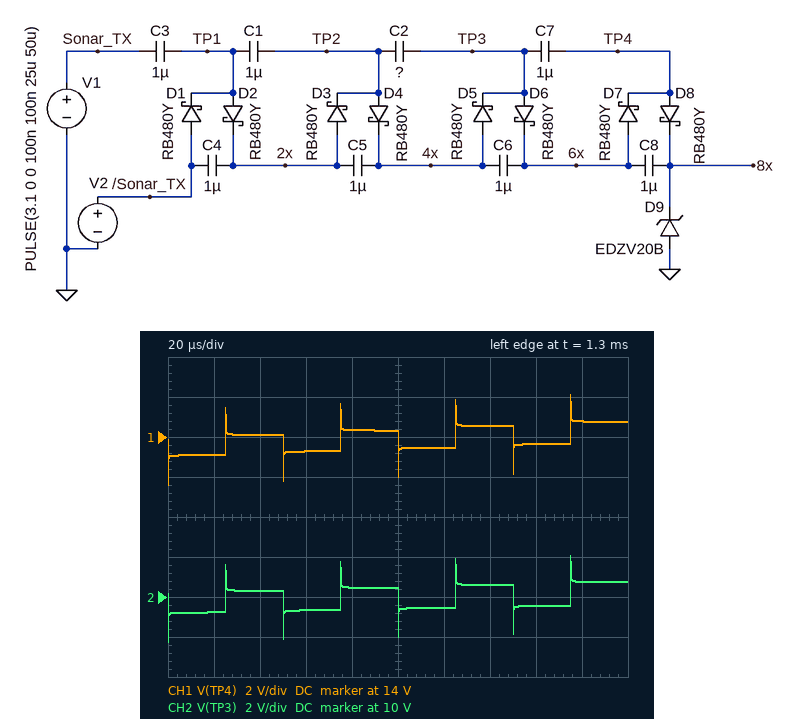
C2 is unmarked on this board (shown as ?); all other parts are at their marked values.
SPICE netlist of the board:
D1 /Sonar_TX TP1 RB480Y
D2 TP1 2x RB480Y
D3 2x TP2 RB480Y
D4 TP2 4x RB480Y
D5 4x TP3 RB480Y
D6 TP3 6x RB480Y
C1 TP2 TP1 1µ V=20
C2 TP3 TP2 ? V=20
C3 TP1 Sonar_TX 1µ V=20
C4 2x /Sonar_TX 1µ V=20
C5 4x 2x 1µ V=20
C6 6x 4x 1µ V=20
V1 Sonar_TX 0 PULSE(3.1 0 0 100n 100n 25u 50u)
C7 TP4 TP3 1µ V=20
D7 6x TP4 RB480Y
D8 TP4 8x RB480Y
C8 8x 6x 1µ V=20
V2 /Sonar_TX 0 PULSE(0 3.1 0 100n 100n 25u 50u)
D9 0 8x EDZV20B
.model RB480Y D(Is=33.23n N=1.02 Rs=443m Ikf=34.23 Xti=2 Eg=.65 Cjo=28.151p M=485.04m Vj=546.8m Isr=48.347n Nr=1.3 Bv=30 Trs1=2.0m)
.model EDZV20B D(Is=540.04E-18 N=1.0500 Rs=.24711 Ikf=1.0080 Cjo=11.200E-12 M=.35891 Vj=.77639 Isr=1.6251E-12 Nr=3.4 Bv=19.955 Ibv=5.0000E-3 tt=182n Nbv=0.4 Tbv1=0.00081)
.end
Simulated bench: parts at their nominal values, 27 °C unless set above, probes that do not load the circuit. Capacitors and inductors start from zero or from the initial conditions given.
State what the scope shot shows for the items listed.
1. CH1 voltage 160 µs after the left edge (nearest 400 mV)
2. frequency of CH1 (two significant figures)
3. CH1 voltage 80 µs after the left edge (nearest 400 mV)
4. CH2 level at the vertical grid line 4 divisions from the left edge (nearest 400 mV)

13.6 V
20 kHz
14.4 V
10.4 V
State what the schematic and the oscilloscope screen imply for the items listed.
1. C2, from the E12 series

10 µF
